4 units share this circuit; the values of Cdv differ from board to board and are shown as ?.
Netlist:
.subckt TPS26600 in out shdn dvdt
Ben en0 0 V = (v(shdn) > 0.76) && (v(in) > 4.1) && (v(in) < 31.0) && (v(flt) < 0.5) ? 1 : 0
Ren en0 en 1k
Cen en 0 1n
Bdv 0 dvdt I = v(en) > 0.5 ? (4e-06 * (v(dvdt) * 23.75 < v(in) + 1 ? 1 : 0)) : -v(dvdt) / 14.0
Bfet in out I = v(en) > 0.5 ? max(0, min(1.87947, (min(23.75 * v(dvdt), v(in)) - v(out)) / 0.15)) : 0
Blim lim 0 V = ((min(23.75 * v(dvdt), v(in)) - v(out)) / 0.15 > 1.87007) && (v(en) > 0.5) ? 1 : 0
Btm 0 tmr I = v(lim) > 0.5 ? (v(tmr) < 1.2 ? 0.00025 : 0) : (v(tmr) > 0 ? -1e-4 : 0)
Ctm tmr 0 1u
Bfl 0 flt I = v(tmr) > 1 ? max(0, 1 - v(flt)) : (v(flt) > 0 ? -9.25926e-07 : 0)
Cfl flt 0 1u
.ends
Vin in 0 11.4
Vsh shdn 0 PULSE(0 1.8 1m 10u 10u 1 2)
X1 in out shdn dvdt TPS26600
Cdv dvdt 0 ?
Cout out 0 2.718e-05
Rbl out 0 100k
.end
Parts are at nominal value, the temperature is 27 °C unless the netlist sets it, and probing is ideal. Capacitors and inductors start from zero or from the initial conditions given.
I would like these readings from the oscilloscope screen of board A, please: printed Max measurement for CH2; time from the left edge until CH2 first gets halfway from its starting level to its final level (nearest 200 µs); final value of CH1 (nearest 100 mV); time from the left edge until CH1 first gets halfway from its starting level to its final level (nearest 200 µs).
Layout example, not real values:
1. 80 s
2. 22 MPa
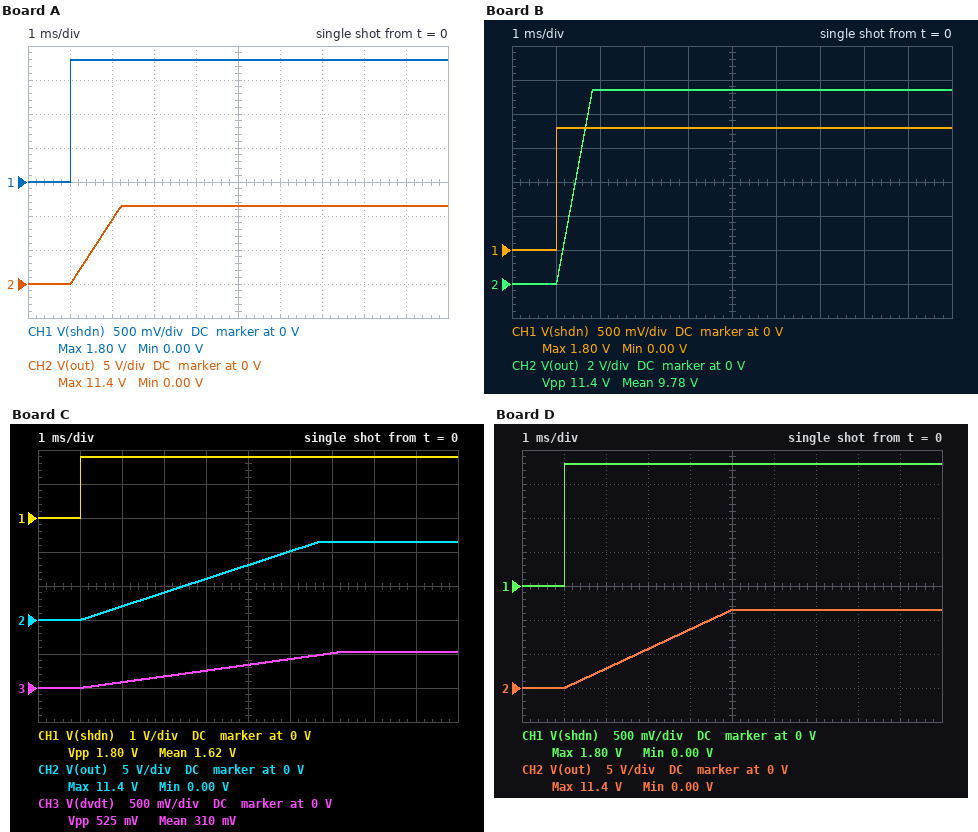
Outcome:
1. 11.4 V
2. 1.6 ms
3. 1.8 V
4. 1.0 ms
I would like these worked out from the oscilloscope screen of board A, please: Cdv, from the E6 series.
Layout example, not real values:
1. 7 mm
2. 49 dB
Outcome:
1. 10 nF
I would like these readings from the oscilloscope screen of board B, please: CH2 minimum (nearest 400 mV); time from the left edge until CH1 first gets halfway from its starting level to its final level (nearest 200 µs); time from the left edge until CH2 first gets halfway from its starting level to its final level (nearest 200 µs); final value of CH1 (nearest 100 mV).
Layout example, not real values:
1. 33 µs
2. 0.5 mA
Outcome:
1. 0 V
2. 1.0 ms
3. 1.4 ms
4. 1.8 V
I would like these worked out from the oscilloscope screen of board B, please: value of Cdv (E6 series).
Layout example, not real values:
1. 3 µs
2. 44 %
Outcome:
1. 6.8 nF
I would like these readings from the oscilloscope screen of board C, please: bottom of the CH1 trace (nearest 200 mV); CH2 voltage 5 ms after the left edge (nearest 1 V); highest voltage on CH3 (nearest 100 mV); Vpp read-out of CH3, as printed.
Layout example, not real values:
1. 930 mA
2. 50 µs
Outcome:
1. 0 V
2. 8 V
3. 500 mV
4. 525 mV
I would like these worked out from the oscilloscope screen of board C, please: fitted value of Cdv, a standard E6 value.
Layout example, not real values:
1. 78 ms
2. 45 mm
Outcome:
1. 47 nF
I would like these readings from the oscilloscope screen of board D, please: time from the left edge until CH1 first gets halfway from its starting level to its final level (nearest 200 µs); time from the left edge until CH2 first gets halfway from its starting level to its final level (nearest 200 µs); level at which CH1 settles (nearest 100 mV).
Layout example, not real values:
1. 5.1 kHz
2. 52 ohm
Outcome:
1. 1.0 ms
2. 3.0 ms
3. 1.8 V
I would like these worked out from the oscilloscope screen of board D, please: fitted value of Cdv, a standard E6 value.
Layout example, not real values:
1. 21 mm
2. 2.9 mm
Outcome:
1. 33 nF
